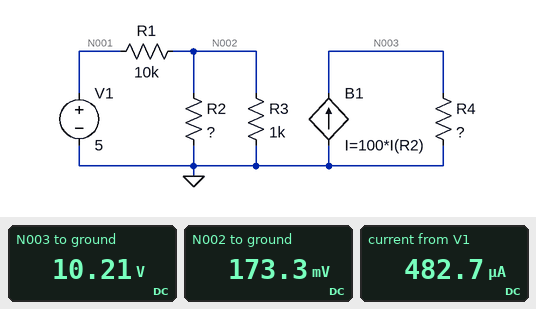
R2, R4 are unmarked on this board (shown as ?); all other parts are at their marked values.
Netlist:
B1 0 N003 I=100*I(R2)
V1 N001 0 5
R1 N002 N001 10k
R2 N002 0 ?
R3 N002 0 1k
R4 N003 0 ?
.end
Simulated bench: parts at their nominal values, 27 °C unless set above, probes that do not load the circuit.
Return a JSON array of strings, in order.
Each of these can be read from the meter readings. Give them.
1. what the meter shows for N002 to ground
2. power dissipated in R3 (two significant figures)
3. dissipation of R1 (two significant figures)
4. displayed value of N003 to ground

["173.3 mV", "30 µW", "2.3 mW", "10.21 V"]
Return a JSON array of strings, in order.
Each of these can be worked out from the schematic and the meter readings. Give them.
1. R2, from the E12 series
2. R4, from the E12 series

["560 Ω", "330 Ω"]
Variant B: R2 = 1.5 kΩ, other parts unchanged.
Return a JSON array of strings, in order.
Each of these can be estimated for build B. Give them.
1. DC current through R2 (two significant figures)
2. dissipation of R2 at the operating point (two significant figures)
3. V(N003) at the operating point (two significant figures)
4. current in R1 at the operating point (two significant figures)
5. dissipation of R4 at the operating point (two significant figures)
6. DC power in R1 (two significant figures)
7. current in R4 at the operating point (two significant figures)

["190 µA", "53 µW", "6.2 V", "470 µA", "120 mW", "2.2 mW", "19 mA"]
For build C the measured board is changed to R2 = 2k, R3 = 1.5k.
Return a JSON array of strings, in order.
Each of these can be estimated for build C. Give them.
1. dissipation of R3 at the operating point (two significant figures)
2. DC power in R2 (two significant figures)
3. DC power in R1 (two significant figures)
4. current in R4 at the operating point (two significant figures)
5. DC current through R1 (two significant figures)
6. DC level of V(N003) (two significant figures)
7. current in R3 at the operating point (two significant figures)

["100 µW", "78 µW", "2.1 mW", "20 mA", "460 µA", "6.5 V", "260 µA"]
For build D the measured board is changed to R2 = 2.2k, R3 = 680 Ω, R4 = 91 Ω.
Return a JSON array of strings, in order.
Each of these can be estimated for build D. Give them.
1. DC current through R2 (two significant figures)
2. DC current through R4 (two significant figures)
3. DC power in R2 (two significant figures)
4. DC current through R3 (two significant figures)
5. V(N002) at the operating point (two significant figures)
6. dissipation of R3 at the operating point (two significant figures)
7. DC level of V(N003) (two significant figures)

["110 µA", "11 mA", "28 µW", "360 µA", "250 mV", "90 µW", "1.0 V"]
